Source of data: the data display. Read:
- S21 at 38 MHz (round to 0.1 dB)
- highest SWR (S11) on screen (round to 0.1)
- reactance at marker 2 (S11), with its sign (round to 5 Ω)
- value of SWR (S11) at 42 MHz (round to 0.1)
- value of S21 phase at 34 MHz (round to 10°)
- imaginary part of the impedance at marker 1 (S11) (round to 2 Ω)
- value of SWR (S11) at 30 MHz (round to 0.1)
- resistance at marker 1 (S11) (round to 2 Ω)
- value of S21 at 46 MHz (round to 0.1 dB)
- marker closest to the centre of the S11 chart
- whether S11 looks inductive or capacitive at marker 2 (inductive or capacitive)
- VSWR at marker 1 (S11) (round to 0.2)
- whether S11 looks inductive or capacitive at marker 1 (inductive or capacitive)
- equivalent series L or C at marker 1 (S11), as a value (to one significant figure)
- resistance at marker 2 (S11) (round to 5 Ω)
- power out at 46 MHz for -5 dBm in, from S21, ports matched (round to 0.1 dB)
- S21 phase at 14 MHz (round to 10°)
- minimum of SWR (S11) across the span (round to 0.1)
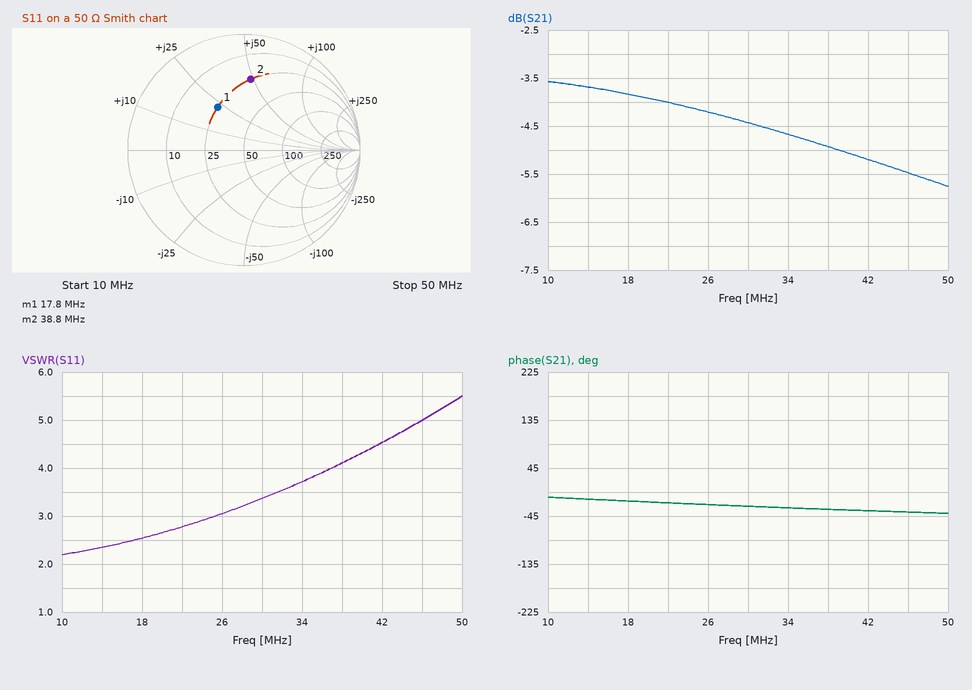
-4.9 dB
5.5
+50 Ω
4.5
-30°
+22 Ω
3.4
24 Ω
-5.5 dB
marker 1
inductive
2.6
inductive
200 nH
25 Ω
-10.5 dBm
-10°
2.2
